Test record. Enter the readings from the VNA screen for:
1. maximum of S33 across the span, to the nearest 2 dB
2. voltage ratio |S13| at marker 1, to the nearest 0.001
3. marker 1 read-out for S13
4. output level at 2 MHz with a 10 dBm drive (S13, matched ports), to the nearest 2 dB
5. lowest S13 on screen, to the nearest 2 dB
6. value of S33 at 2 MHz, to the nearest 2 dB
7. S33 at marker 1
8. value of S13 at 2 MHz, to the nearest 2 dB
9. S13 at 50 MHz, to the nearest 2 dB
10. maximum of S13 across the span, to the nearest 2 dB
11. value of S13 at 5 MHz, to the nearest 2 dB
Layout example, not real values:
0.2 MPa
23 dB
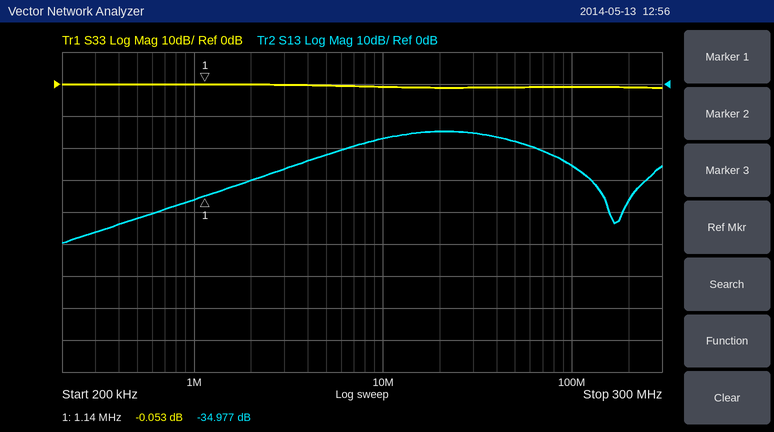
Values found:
0 dB
0.018
-34.977 dB
-20 dBm
-50 dB
0 dB
-0.053 dB
-30 dB
-18 dB
-14 dB
-22 dB
